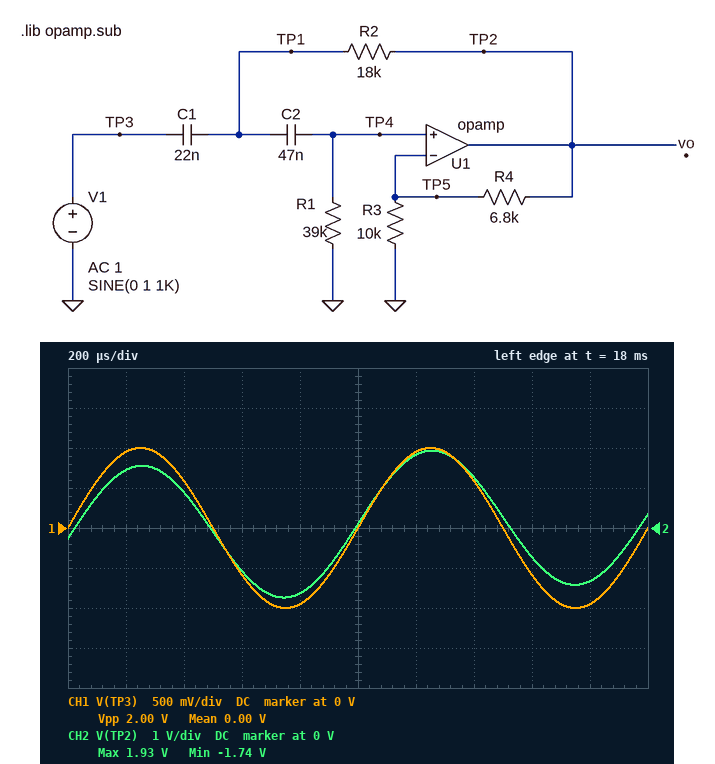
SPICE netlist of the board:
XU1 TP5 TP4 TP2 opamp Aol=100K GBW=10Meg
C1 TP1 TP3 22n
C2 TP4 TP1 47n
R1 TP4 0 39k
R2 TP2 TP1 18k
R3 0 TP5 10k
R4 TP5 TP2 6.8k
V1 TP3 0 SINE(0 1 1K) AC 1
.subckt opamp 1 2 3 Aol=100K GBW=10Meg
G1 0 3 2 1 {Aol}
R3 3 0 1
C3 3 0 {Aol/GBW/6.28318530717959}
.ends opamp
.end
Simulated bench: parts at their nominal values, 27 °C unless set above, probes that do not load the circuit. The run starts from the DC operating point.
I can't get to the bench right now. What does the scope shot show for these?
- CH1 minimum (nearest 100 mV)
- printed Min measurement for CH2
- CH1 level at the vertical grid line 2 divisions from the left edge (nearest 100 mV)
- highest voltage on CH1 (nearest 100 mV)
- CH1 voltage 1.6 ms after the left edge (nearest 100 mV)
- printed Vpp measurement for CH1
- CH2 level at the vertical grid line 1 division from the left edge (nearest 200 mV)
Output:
-1.0 V
-1.74 V
600 mV
1.0 V
-600 mV
2.00 V
1.4 V
